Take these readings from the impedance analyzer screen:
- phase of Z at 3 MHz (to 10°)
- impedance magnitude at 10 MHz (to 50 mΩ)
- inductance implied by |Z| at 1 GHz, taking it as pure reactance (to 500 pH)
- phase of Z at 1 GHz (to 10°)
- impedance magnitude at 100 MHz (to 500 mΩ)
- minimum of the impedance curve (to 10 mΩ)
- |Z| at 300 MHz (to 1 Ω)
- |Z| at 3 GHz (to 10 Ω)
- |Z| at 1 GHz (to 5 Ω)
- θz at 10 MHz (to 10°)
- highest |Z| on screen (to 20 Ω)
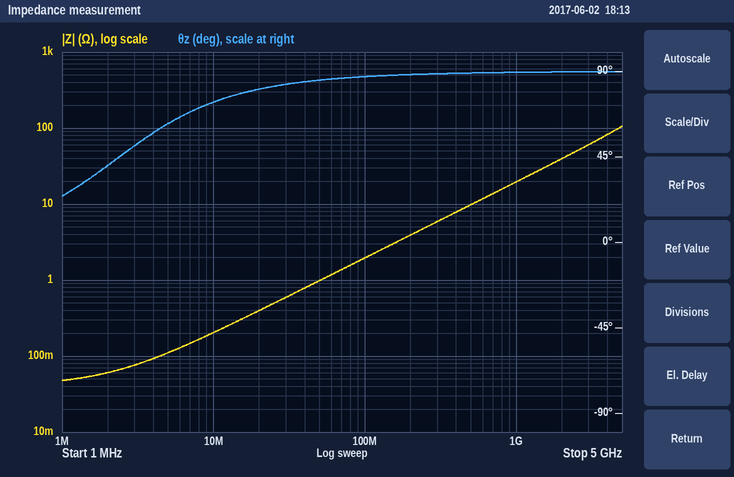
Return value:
50°
200 mΩ
3.0 nH
90°
2.0 Ω
50 mΩ
6 Ω
60 Ω
20 Ω
70°
100 Ω
